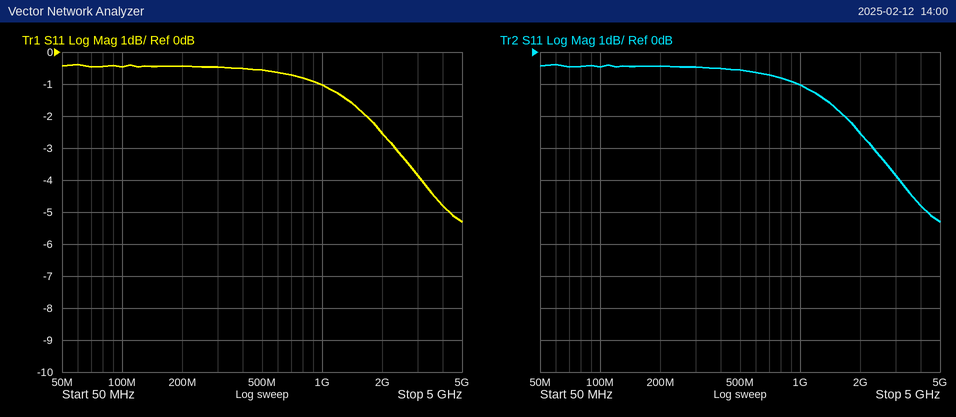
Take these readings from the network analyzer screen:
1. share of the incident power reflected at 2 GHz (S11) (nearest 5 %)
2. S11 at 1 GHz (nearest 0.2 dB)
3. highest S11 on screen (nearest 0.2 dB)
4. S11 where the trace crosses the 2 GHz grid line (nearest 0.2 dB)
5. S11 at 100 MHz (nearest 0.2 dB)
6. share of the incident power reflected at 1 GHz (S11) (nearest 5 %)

55 %
-1.0 dB
-0.4 dB
-2.6 dB
-0.4 dB
80 %
